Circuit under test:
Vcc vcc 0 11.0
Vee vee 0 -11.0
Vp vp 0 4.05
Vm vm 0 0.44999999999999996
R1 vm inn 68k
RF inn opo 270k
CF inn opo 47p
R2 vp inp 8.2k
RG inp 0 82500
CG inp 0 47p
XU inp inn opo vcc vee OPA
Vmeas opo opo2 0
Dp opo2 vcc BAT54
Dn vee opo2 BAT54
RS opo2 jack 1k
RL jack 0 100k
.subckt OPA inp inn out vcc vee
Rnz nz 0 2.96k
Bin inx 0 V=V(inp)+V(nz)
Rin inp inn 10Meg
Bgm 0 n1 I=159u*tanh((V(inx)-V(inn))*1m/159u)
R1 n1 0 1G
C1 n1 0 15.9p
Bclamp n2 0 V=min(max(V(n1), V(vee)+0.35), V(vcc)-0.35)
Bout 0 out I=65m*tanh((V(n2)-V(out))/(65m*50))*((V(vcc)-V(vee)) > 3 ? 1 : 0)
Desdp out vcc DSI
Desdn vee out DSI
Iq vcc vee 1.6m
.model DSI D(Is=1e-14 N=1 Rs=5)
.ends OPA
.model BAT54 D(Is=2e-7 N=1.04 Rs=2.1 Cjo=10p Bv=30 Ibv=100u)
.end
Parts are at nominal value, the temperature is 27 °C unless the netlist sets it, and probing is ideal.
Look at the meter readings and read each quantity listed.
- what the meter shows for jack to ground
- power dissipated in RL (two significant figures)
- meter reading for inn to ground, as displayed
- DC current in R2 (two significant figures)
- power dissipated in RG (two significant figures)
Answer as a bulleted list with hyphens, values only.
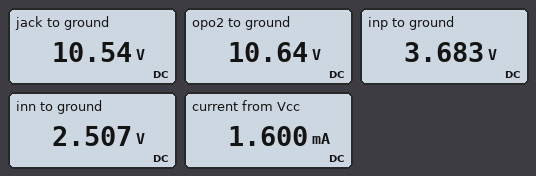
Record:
- 10.54 V
- 1.1 mW
- 2.507 V
- 45 µA
- 160 µW
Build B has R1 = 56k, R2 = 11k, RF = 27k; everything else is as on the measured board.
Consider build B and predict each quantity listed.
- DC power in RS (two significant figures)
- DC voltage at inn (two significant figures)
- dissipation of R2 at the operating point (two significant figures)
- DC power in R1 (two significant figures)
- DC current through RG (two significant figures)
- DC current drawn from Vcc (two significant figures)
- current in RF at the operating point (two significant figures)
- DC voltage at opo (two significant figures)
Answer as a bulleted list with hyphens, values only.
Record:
- 2.5 µW
- 3.6 V
- 21 µW
- 170 µW
- 43 µA
- 1.6 mA
- 56 µA
- 5.1 V
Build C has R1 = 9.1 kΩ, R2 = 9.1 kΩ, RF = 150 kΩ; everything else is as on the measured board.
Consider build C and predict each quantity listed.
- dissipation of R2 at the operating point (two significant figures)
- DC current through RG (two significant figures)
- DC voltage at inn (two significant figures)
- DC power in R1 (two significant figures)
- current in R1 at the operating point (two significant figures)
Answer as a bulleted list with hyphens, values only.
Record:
- 18 µW
- 44 µA
- 1.0 V
- 38 µW
- 64 µA
